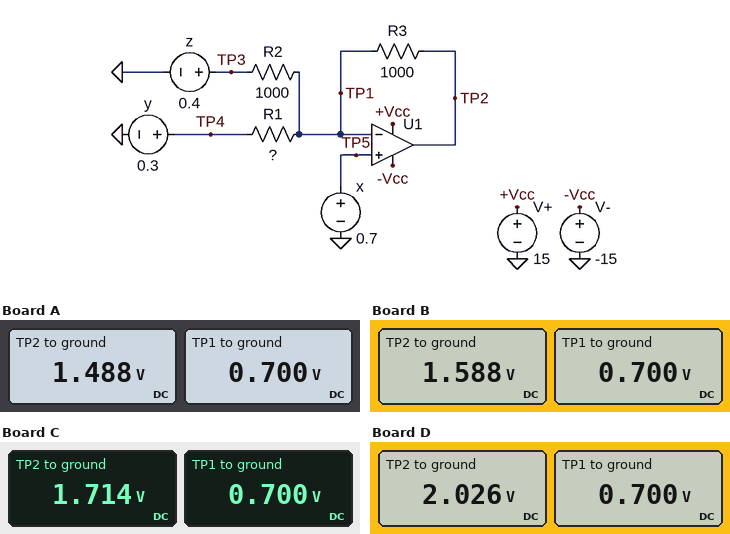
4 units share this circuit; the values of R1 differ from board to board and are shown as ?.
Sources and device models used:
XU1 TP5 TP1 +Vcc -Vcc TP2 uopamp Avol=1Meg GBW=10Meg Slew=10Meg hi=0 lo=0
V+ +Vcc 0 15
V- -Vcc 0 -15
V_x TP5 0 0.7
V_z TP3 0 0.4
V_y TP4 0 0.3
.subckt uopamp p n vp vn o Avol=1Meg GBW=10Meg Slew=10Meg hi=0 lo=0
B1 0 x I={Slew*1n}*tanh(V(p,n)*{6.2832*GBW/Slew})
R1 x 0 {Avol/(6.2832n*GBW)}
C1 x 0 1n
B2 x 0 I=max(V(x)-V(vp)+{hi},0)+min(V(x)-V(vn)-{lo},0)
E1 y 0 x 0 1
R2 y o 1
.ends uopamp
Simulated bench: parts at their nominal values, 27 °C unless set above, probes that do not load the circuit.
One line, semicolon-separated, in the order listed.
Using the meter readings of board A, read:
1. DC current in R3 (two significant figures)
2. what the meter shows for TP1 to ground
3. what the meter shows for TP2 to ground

790 µA; 0.700 V; 1.488 V
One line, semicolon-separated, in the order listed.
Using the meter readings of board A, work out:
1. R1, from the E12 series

820 Ω
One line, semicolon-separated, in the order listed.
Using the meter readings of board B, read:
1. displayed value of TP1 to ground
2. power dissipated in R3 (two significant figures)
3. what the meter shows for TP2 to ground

0.700 V; 790 µW; 1.588 V
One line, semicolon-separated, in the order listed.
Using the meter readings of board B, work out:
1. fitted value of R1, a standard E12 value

680 Ω
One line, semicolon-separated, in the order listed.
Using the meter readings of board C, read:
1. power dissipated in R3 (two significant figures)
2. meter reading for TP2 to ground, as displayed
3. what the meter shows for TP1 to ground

1.0 mW; 1.714 V; 0.700 V
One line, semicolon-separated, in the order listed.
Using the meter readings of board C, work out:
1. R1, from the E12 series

560 Ω
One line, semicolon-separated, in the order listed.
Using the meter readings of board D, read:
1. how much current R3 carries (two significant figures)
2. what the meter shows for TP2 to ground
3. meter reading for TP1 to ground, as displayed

1.3 mA; 2.026 V; 0.700 V
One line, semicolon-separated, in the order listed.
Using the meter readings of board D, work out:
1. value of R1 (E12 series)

390 Ω
